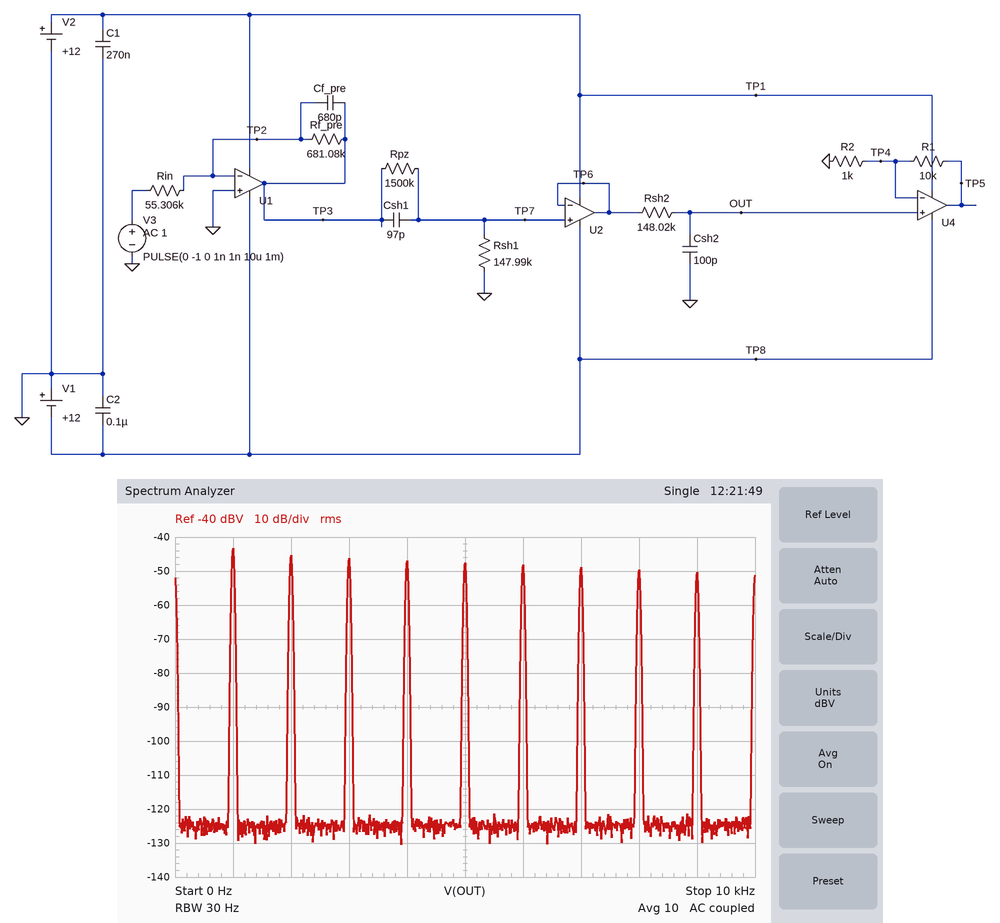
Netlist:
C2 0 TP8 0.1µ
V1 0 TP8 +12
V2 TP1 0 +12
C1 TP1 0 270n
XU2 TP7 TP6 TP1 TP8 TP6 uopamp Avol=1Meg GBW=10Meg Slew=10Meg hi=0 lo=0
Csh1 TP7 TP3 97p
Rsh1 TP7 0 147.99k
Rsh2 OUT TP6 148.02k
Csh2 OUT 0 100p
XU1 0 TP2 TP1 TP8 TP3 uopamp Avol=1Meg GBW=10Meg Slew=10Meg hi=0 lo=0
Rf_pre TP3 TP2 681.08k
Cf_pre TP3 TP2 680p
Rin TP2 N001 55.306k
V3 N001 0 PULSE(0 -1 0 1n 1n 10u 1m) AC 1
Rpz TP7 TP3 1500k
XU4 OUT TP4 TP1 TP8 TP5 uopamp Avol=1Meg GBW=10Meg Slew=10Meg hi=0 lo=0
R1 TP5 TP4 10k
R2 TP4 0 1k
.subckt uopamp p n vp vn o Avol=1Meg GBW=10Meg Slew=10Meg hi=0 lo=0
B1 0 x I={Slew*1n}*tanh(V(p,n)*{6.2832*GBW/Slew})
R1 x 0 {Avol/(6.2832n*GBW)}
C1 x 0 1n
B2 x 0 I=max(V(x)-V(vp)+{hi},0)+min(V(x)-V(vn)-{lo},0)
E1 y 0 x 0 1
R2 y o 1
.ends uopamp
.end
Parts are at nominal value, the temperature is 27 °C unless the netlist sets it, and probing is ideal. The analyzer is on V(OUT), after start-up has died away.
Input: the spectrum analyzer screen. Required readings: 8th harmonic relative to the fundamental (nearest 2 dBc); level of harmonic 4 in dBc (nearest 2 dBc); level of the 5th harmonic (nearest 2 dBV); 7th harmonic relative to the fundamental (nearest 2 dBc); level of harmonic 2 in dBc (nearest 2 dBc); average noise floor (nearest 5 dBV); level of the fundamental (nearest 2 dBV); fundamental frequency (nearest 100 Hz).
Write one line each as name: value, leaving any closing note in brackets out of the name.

8th harmonic relative to the fundamental: -6 dBc
level of harmonic 4 in dBc: -4 dBc
level of the 5th harmonic: -48 dBV
7th harmonic relative to the fundamental: -6 dBc
level of harmonic 2 in dBc: -2 dBc
average noise floor: -125 dBV
level of the fundamental: -44 dBV
fundamental frequency: 1.0 kHz
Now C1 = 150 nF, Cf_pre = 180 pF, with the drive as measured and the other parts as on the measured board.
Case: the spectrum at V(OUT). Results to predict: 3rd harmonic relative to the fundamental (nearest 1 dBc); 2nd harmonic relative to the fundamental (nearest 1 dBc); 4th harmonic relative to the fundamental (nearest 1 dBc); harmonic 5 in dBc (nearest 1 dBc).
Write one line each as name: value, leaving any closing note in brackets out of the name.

3rd harmonic relative to the fundamental: 0 dBc
2nd harmonic relative to the fundamental: 0 dBc
4th harmonic relative to the fundamental: 0 dBc
harmonic 5 in dBc: -1 dBc
